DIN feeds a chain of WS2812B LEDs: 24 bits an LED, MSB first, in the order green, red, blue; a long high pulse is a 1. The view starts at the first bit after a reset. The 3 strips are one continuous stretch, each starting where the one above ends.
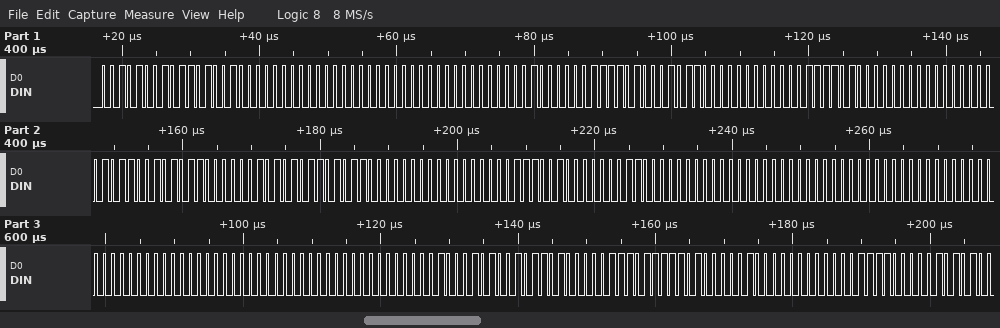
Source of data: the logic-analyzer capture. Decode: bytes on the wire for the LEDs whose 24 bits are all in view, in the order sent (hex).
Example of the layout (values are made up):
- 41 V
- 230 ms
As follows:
- 29 69 00 00 00 00 20 7A 2C 00 3D 00 00 59 58 15 6B 00 00 72 03 00 00 00 00 00 00 00 00 00 00 45 2D 07 7D 04 00 3C 15
